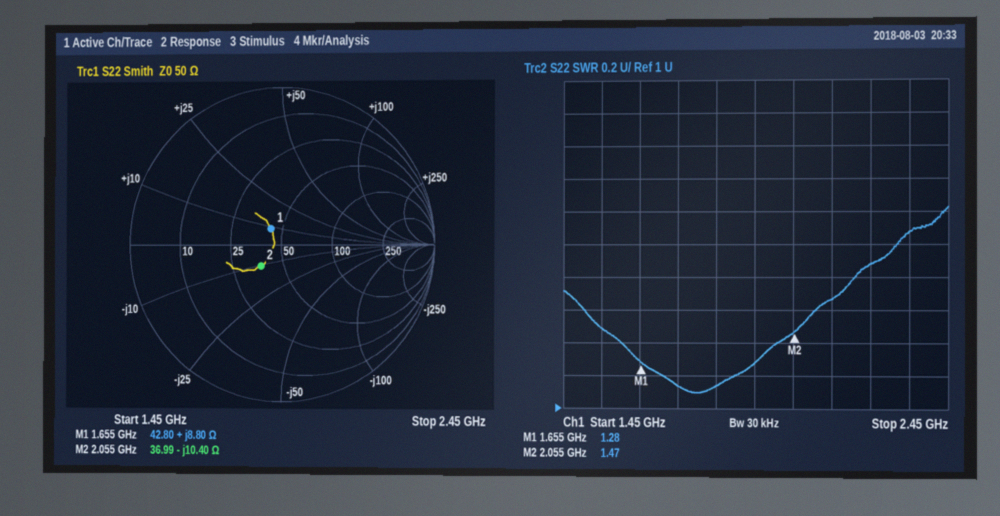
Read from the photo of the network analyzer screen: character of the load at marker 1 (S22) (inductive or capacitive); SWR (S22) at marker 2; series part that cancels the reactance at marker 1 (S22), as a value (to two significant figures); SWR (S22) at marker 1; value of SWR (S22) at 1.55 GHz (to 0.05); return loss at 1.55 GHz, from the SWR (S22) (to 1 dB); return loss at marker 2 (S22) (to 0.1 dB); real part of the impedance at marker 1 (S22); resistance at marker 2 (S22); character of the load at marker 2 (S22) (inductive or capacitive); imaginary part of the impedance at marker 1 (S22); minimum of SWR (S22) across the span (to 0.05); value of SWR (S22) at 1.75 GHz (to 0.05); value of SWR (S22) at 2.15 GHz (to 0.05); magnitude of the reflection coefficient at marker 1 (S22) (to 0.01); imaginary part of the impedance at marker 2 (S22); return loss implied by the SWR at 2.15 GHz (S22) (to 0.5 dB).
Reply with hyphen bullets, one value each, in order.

- inductive
- 1.47
- 11 pF
- 1.28
- 1.50
- 14 dB
- 14.4 dB
- 42.80 Ω
- 36.99 Ω
- capacitive
- +8.80 Ω
- 1.10
- 1.15
- 1.65
- 0.12
- -10.40 Ω
- 12.0 dB
